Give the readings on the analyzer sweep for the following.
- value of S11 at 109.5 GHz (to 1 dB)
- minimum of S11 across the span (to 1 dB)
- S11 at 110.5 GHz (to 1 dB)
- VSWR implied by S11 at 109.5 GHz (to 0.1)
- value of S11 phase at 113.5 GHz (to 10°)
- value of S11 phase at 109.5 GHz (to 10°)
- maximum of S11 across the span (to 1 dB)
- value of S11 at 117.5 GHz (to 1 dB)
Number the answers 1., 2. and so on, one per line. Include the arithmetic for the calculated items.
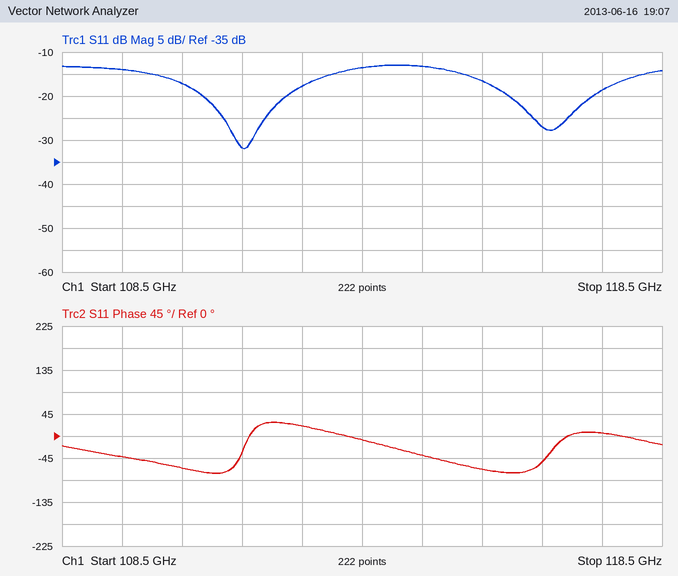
1. -14 dB
2. -32 dB
3. -17 dB
4. |Γ| = 10^(-14/20) = 0.1995; VSWR = (1 + 0.1995)/(1 − 0.1995) ≈ 1.5
5. -10°
6. -40°
7. -13 dB
8. -19 dB
